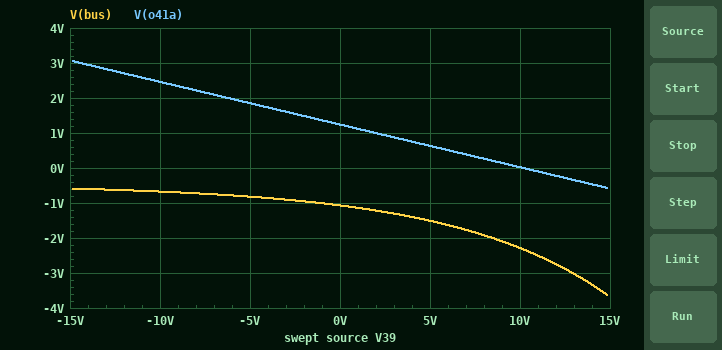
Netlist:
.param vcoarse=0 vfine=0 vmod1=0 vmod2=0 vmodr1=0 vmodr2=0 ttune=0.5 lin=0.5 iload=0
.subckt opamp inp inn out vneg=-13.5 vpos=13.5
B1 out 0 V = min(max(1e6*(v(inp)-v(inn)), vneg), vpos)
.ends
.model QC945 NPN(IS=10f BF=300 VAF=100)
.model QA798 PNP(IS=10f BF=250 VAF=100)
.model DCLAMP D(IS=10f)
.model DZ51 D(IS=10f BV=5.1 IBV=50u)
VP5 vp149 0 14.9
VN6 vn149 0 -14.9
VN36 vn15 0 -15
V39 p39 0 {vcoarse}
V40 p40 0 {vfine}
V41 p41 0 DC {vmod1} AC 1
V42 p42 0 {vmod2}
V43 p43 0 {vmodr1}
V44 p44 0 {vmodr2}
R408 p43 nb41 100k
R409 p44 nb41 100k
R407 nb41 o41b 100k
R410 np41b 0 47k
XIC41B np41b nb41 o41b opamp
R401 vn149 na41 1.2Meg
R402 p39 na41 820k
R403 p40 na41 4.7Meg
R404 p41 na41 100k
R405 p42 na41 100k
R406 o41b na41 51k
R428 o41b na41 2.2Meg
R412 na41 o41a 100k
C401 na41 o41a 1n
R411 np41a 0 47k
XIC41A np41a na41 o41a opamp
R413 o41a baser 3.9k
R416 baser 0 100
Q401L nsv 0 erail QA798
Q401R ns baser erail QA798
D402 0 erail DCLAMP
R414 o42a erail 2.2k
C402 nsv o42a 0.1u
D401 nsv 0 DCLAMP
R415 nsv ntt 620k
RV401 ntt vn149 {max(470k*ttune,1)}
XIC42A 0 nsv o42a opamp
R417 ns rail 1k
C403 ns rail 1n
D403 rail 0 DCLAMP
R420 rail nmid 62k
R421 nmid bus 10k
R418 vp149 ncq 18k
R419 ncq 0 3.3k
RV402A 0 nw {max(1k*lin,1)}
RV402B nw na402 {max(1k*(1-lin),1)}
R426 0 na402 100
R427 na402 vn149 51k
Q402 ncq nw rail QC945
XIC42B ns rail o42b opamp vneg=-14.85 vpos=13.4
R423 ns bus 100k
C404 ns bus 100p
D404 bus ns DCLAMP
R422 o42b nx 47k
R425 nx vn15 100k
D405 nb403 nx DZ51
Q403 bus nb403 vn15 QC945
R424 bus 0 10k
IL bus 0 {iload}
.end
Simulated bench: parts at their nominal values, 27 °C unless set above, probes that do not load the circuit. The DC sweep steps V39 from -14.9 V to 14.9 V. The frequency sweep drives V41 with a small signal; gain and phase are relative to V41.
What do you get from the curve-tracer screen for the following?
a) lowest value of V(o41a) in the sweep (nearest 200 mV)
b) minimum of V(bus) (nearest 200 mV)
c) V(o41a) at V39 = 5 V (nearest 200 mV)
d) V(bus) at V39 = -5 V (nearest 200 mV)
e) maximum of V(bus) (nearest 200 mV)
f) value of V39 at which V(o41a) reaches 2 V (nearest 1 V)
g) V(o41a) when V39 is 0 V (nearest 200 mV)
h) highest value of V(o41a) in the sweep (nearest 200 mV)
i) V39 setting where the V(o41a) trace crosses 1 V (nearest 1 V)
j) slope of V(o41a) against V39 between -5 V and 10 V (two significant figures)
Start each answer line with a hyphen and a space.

- -600 mV
- -3.6 V
- 600 mV
- -800 mV
- -600 mV
- -6 V
- 1.2 V
- 3.0 V
- 2 V
- -0.12 V/V
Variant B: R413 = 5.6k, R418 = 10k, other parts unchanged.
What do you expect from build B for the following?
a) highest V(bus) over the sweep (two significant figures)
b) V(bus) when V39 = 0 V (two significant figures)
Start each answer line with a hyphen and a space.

- -740 mV
- -1.3 V
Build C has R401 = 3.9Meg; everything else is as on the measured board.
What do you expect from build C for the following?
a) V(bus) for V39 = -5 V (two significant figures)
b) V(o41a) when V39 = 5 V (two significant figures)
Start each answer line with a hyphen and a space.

- -1.2 V
- -230 mV
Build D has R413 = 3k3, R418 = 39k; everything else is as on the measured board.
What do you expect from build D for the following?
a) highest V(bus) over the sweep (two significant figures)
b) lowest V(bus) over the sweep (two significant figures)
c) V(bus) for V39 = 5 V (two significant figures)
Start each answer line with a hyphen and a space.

- -540 mV
- -4.0 V
- -1.4 V
